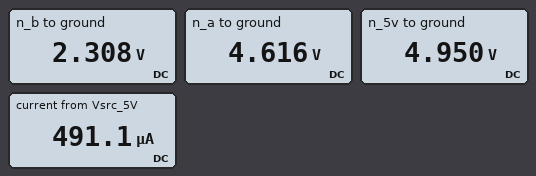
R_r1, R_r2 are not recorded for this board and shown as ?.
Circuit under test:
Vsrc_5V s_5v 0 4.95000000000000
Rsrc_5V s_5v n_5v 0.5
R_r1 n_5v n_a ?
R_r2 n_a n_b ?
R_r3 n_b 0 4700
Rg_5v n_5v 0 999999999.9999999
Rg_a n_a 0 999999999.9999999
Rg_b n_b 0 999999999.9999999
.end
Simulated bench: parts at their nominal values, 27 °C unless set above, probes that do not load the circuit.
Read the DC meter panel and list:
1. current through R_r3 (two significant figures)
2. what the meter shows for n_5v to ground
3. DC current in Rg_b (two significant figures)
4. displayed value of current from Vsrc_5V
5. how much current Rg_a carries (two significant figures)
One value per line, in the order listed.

490 µA
4.950 V
2.3 nA
491.1 µA
4.6 nA
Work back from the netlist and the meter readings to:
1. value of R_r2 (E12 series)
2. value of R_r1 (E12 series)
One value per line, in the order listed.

4.7 kΩ
680 Ω
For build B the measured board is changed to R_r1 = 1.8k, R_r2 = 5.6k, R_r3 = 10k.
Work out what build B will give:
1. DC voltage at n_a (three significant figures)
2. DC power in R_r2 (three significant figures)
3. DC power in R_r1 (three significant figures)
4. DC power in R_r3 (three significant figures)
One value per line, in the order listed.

4.44 V
453 µW
146 µW
809 µW
